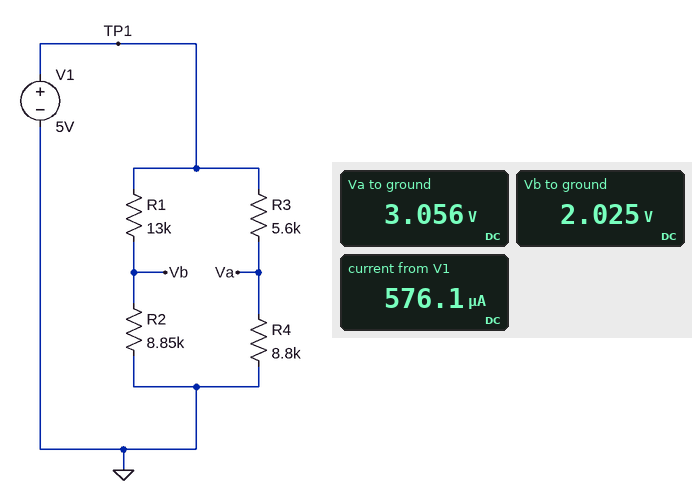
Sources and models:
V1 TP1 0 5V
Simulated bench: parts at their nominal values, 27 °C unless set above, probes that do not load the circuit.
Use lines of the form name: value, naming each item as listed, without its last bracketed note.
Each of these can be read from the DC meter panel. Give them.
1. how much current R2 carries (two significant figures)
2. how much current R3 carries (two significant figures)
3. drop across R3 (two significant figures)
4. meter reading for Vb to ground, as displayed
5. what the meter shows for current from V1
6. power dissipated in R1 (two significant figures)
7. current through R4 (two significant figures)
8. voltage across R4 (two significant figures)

how much current R2 carries: 230 µA
how much current R3 carries: 350 µA
drop across R3: 1.9 V
meter reading for Vb to ground, as displayed: 2.025 V
what the meter shows for current from V1: 576.1 µA
power dissipated in R1: 680 µW
current through R4: 350 µA
voltage across R4: 3.1 V
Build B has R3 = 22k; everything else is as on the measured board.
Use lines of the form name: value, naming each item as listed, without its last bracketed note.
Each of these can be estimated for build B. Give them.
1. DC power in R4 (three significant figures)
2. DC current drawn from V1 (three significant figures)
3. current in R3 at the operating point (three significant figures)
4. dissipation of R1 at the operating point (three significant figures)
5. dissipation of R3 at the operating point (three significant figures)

DC power in R4: 232 µW
DC current drawn from V1: 391 µA
current in R3 at the operating point: 162 µA
dissipation of R1 at the operating point: 681 µW
dissipation of R3 at the operating point: 580 µW
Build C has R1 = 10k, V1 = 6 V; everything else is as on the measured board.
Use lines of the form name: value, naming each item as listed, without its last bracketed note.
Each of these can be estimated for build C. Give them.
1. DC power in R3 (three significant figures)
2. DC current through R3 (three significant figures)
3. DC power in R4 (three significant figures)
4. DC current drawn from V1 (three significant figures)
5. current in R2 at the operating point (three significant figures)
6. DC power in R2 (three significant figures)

DC power in R3: 972 µW
DC current through R3: 417 µA
DC power in R4: 1.53 mW
DC current drawn from V1: 735 µA
current in R2 at the operating point: 318 µA
DC power in R2: 897 µW
